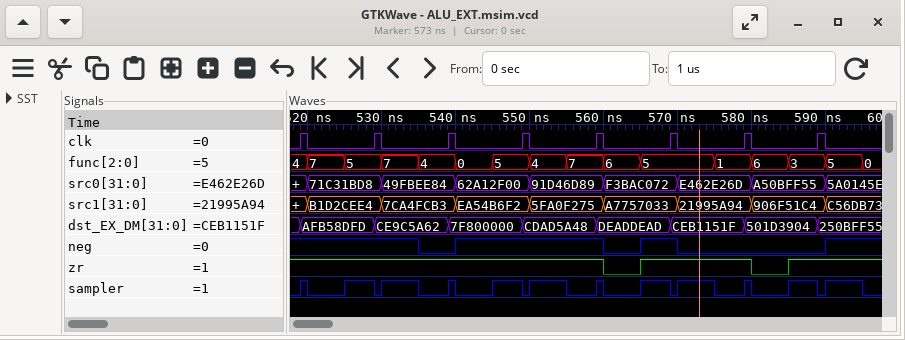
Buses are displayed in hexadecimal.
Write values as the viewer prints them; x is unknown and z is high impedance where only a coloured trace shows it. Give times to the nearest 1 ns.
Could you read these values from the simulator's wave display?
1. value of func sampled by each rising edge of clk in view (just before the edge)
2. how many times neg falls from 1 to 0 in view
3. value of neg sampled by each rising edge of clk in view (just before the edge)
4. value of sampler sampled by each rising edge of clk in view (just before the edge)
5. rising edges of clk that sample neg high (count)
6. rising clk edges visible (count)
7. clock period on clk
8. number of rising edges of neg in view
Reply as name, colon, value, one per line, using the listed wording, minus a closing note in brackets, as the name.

value of func sampled by each rising edge of clk in view: 4, 5, 4, 5, 7, 5, 1, 3
how many times neg falls from 1 to 0 in view: 3
value of neg sampled by each rising edge of clk in view: 1 1 0 1 1 1 0 0
value of sampler sampled by each rising edge of clk in view: 0 1 0 1 0 1 0 1
rising edges of clk that sample neg high: 5
rising clk edges visible: 8
clock period on clk: 10 ns
number of rising edges of neg in view: 3
